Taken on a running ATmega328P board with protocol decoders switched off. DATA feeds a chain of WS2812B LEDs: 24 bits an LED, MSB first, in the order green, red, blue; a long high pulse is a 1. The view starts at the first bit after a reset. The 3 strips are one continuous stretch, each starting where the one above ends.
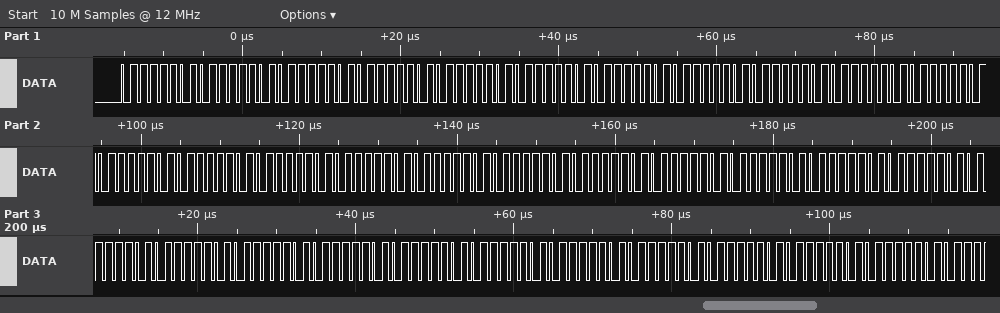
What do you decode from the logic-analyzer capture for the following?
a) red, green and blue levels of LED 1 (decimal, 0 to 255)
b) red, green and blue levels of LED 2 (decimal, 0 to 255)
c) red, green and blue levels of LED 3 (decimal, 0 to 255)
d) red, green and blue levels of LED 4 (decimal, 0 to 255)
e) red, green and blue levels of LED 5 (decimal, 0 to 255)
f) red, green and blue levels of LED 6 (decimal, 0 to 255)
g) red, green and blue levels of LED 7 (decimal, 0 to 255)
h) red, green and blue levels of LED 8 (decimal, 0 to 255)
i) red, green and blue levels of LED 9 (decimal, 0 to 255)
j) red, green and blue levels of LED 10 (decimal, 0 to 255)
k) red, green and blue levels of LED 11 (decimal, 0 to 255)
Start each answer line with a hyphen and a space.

- 125, 125, 125
- 125, 125, 125
- 125, 125, 125
- 125, 125, 125
- 125, 125, 125
- 125, 125, 125
- 125, 125, 125
- 125, 125, 125
- 125, 125, 125
- 125, 125, 125
- 125, 125, 125
